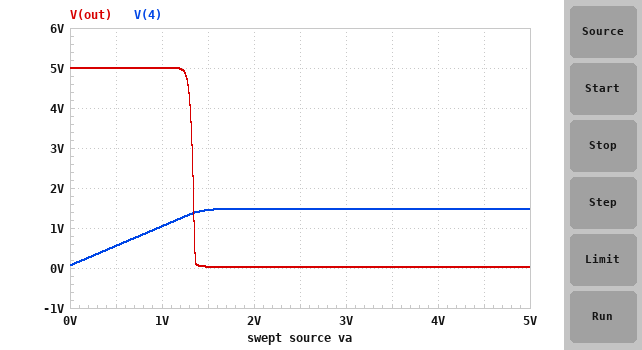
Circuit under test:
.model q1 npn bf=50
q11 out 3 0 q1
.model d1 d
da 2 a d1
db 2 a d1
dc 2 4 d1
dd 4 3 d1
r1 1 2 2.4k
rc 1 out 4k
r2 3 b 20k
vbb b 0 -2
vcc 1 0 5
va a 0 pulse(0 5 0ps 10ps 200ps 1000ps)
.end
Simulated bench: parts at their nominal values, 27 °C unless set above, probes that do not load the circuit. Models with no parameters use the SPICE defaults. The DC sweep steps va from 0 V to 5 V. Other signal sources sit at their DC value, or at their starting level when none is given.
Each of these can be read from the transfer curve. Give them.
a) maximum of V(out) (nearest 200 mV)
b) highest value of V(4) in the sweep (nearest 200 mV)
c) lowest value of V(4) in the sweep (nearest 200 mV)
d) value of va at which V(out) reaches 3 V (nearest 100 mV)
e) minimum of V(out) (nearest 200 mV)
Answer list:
5.0 V
1.4 V
0 V
1.3 V
0 V
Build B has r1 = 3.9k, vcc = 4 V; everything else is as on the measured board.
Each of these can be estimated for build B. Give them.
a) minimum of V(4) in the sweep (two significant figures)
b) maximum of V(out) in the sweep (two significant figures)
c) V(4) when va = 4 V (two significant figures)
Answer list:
44 mV
4.0 V
1.4 V
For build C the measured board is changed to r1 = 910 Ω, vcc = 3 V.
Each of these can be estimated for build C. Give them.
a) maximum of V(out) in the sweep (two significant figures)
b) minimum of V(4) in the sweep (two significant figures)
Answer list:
3.0 V
73 mV
